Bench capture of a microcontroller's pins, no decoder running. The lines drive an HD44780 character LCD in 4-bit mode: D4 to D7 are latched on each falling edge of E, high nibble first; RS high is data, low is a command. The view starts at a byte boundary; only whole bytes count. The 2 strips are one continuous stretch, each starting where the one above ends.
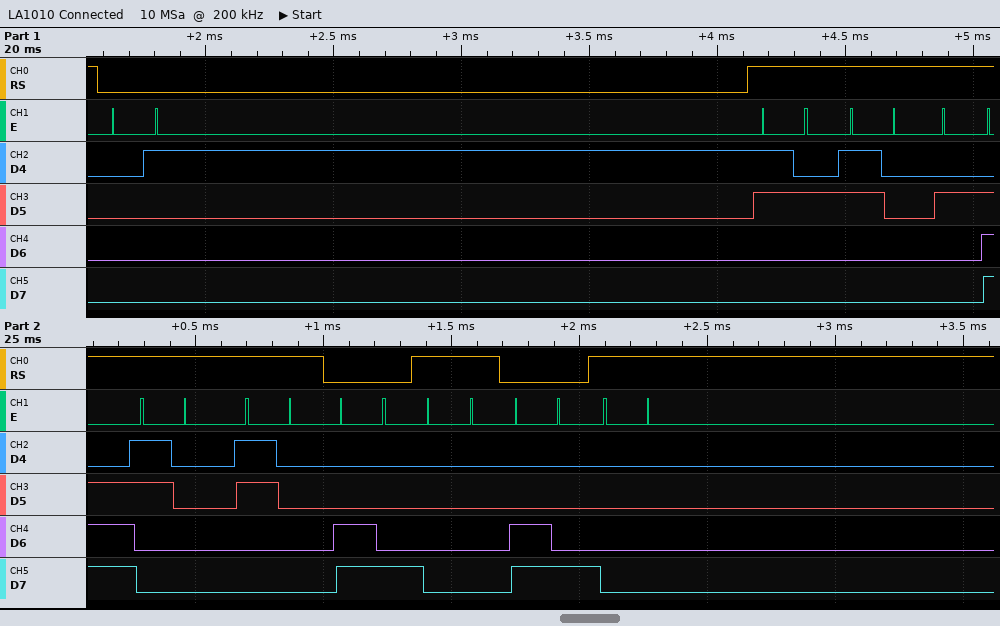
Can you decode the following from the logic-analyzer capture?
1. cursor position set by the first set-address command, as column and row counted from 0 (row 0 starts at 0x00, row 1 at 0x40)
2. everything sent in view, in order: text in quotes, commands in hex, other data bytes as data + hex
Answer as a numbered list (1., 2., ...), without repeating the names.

1. column 8, row 1
2. 0x01 "20.00" 0xC8 data 00 0xC8 data 00
